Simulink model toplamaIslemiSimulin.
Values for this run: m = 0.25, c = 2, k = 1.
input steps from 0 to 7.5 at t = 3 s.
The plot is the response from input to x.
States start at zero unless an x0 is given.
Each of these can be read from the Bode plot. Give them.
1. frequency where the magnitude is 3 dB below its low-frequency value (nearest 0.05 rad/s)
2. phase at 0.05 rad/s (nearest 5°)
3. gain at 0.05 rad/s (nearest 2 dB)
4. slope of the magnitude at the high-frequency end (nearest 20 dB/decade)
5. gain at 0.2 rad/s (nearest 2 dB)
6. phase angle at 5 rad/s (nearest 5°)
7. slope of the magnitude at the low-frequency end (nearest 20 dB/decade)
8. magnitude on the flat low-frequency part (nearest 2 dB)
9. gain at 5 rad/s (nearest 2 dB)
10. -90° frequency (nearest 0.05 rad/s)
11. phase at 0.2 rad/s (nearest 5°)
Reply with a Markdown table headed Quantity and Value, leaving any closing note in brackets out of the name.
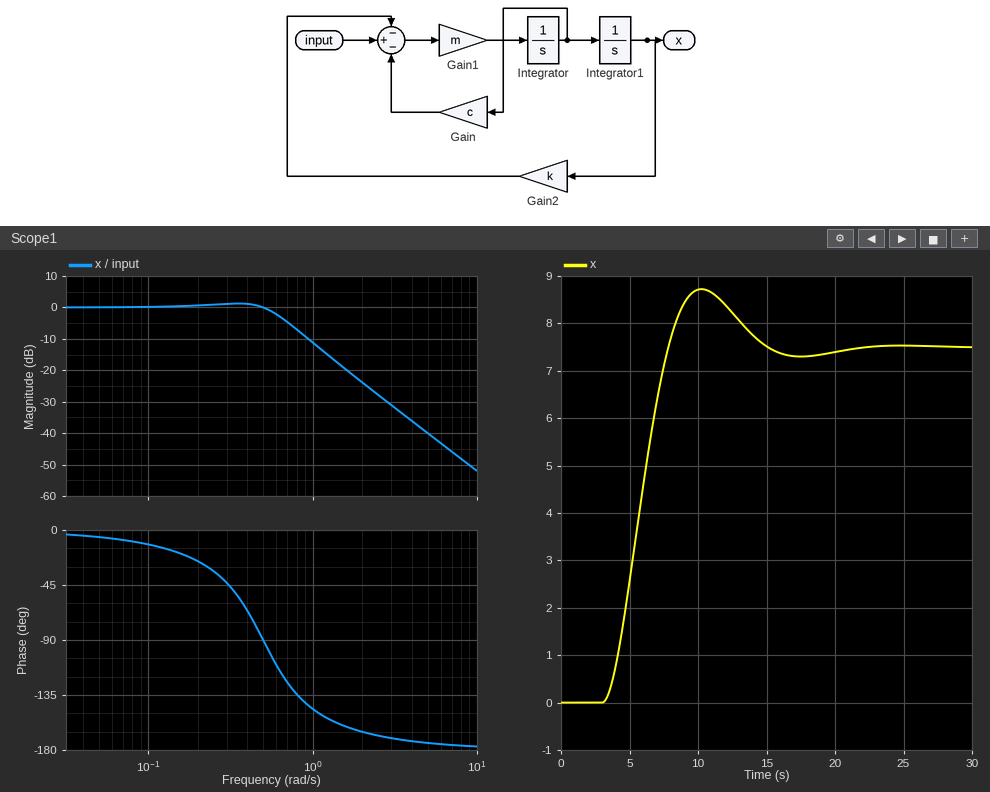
| Quantity | Value |
|---|---|
| frequency where the magnitude is 3 dB below its low-frequency value | 0.65 rad/s |
| phase at 0.05 rad/s | -5° |
| gain at 0.05 rad/s | 0 dB |
| slope of the magnitude at the high-frequency end | -40 dB/decade |
| gain at 0.2 rad/s | 0 dB |
| phase angle at 5 rad/s | -175° |
| slope of the magnitude at the low-frequency end | 0 dB/decade |
| magnitude on the flat low-frequency part | 0 dB |
| gain at 5 rad/s | -40 dB |
| -90° frequency | 0.50 rad/s |
| phase at 0.2 rad/s | -25° |
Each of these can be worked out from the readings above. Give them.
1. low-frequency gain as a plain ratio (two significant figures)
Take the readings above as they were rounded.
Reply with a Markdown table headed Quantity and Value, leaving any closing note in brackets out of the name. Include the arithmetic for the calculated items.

| Quantity | Value |
|---|---|
| low-frequency gain as a plain ratio | 10^(0 / 20) = 1.0 |
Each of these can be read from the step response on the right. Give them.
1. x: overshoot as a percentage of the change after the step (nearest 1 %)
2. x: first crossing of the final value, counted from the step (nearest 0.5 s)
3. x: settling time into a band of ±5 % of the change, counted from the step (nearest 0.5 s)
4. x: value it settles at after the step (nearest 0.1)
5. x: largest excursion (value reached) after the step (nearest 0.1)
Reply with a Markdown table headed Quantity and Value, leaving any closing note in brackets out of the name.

| Quantity | Value |
|---|---|
| x: overshoot as a percentage of the change after the step | 16 % |
| x: first crossing of the final value, counted from the step | 5.0 s |
| x: settling time into a band of ±5 % of the change, counted from the step | 10.5 s |
| x: value it settles at after the step | 7.5 |
| x: largest excursion (value reached) after the step | 8.7 |
